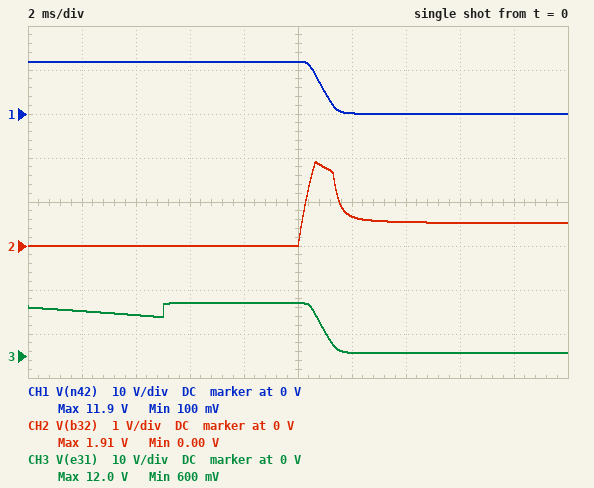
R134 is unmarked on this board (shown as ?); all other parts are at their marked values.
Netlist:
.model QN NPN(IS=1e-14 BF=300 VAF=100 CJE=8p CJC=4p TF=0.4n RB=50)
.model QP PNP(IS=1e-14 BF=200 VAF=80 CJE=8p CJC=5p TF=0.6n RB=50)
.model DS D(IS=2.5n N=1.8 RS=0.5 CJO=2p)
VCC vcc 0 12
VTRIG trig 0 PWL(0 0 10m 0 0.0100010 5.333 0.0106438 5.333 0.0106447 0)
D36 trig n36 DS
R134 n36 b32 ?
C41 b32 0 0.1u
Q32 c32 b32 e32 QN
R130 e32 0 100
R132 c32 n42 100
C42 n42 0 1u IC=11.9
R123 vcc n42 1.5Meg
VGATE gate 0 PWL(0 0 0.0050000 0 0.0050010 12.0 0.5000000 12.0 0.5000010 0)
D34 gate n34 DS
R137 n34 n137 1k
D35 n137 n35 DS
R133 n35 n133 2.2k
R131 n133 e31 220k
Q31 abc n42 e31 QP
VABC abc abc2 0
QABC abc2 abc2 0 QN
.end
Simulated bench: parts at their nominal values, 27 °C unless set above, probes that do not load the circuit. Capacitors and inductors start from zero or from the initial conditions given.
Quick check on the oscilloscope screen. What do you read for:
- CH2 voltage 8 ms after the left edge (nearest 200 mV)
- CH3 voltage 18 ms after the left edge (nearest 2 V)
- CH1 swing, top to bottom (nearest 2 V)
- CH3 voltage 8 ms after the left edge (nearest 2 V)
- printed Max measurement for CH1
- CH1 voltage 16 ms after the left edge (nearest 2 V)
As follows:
0 V
0 V
12 V
12 V
11.9 V
0 V
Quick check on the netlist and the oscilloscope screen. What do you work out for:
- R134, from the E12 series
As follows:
12 kΩ
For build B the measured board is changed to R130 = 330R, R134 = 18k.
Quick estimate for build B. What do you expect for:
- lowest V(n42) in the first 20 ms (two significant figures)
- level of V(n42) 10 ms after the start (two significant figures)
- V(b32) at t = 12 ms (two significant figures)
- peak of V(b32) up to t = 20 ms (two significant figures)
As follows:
64 mV
12 V
1.3 V
1.4 V
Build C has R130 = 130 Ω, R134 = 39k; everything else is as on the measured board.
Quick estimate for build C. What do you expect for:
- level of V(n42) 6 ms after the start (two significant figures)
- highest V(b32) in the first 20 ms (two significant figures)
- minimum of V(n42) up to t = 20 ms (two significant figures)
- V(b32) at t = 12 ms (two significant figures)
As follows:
12 V
730 mV
8.5 V
710 mV
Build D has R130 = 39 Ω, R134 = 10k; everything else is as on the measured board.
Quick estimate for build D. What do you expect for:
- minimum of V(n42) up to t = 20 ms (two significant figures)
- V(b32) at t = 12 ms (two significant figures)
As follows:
55 mV
570 mV
